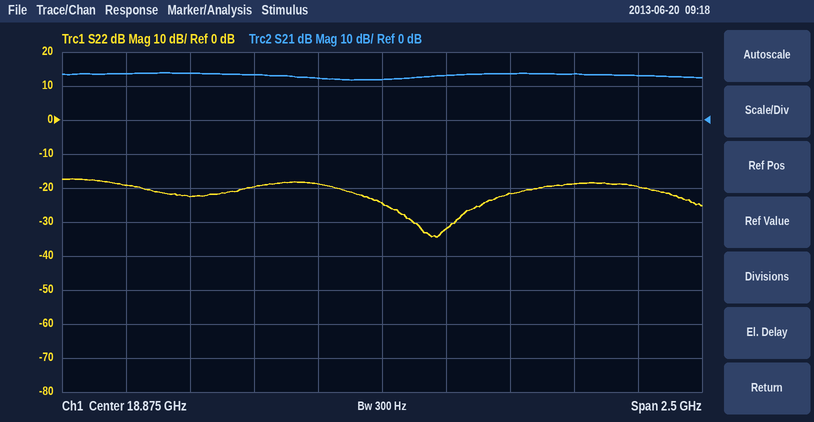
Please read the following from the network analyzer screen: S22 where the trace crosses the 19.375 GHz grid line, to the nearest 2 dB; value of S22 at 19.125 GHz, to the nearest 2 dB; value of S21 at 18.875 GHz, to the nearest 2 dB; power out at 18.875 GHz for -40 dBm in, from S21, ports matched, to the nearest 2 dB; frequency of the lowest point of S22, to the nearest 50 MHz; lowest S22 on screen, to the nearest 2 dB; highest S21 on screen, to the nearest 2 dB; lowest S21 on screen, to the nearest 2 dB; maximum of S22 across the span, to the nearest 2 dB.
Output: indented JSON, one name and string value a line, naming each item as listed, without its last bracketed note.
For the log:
{
  "S22 where the trace crosses the 19.375 GHz grid line, to the nearest 2 dB": "-22 dB",
  "value of S22 at 19.125 GHz, to the nearest 2 dB": "-32 dB",
  "value of S21 at 18.875 GHz, to the nearest 2 dB": "12 dB",
  "power out at 18.875 GHz for -40 dBm in, from S21, ports matched, to the nearest 2 dB": "-28 dBm",
  "frequency of the lowest point of S22, to the nearest 50 MHz": "19.10 GHz",
  "lowest S22 on screen, to the nearest 2 dB": "-34 dB",
  "highest S21 on screen, to the nearest 2 dB": "14 dB",
  "lowest S21 on screen, to the nearest 2 dB": "12 dB",
  "maximum of S22 across the span, to the nearest 2 dB": "-18 dB"
}
